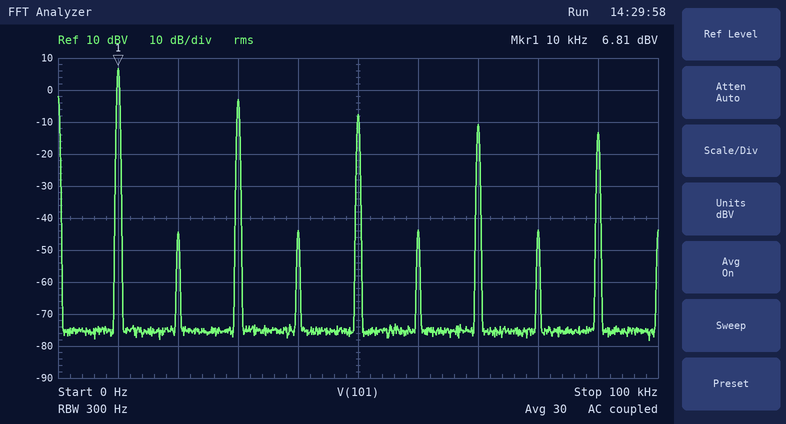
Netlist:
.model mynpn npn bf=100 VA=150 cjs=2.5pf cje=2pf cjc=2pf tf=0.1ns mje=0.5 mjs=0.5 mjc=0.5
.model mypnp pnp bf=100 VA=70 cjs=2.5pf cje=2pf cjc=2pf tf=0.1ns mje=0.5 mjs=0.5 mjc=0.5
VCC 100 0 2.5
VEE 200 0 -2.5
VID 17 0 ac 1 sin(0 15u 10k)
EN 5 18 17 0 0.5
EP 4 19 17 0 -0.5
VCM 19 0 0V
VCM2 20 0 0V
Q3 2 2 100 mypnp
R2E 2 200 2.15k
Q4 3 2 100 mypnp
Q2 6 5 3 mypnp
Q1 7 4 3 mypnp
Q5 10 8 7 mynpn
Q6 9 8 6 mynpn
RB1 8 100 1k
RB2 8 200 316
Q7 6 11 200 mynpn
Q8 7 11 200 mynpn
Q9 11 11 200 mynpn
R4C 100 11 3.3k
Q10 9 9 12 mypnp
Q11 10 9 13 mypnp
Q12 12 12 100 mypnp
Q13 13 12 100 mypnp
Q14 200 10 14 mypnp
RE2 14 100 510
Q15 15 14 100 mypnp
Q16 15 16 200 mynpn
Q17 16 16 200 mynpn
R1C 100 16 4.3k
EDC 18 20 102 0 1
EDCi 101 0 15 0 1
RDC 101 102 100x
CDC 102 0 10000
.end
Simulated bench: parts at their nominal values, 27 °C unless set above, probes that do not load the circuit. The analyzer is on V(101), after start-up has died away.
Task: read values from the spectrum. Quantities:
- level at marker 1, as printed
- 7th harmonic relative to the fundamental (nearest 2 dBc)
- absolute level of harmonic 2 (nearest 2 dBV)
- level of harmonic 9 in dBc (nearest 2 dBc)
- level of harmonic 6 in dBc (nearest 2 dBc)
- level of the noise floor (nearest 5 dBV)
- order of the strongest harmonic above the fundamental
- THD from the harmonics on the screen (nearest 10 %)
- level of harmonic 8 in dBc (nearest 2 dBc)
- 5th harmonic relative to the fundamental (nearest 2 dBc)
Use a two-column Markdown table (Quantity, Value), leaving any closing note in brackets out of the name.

| Quantity | Value |
|---|---|
| level at marker 1, as printed | 6.81 dBV |
| 7th harmonic relative to the fundamental | -18 dBc |
| absolute level of harmonic 2 | -44 dBV |
| level of harmonic 9 in dBc | -20 dBc |
| level of harmonic 6 in dBc | -50 dBc |
| level of the noise floor | -75 dBV |
| order of the strongest harmonic above the fundamental | 3 |
| THD from the harmonics on the screen | 40 % |
| level of harmonic 8 in dBc | -50 dBc |
| 5th harmonic relative to the fundamental | -14 dBc |
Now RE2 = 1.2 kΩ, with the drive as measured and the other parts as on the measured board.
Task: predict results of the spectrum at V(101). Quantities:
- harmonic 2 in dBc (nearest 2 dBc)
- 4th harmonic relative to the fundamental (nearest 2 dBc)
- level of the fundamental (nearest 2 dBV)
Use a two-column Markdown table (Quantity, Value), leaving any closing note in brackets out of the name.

| Quantity | Value |
|---|---|
| harmonic 2 in dBc | -54 dBc |
| 4th harmonic relative to the fundamental | -56 dBc |
| level of the fundamental | 6 dBV |
